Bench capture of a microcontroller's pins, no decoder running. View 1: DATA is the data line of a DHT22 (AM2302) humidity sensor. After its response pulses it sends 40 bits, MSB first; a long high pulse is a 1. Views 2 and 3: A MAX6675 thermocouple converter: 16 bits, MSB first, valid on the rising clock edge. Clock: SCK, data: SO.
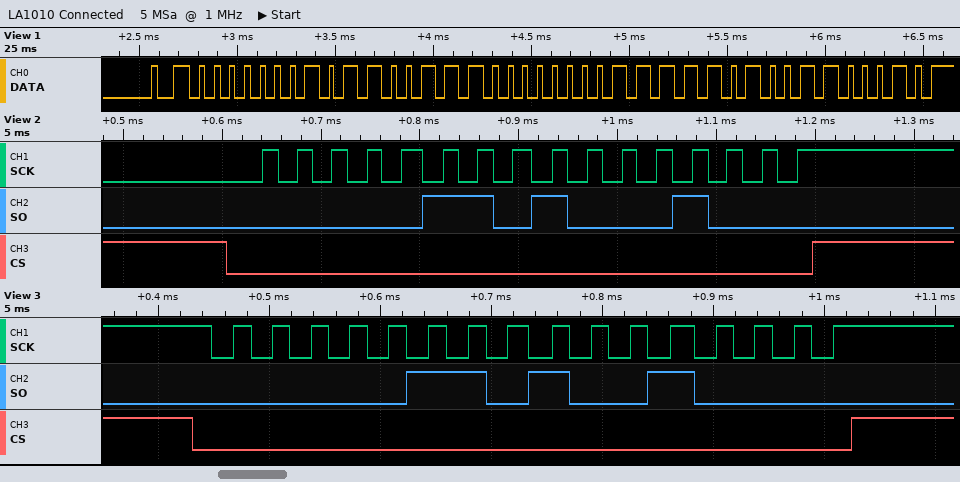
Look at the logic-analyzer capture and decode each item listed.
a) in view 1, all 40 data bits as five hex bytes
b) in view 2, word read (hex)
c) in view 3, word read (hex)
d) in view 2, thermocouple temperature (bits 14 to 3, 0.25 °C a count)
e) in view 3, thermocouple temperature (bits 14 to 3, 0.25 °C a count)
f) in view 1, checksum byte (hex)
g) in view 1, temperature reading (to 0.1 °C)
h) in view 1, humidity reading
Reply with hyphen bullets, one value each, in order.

- 01 67 00 FA 62
- 0x0688
- 0x0690
- 52.25 °C
- 52.50 °C
- 0x62
- 25.0 °C
- 35.9 %
